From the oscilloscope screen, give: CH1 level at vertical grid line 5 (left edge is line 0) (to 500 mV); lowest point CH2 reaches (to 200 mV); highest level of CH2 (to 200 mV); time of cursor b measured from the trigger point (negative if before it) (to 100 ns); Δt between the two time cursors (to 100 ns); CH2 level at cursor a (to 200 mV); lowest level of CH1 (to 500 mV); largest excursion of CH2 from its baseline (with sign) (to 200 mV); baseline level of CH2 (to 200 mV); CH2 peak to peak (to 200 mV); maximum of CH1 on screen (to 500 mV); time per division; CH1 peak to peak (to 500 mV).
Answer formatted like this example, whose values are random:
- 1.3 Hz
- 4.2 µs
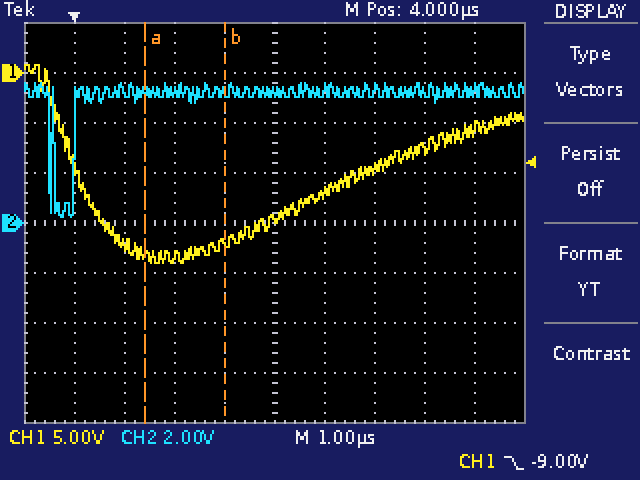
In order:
- -14.5 V
- 200 mV
- 5.6 V
- +3.0 µs
- 1.6 µs
- 5.2 V
- -19.0 V
- -5.0 V
- 5.2 V
- 5.4 V
- 1.0 V
- 1 µs
- 20.0 V
